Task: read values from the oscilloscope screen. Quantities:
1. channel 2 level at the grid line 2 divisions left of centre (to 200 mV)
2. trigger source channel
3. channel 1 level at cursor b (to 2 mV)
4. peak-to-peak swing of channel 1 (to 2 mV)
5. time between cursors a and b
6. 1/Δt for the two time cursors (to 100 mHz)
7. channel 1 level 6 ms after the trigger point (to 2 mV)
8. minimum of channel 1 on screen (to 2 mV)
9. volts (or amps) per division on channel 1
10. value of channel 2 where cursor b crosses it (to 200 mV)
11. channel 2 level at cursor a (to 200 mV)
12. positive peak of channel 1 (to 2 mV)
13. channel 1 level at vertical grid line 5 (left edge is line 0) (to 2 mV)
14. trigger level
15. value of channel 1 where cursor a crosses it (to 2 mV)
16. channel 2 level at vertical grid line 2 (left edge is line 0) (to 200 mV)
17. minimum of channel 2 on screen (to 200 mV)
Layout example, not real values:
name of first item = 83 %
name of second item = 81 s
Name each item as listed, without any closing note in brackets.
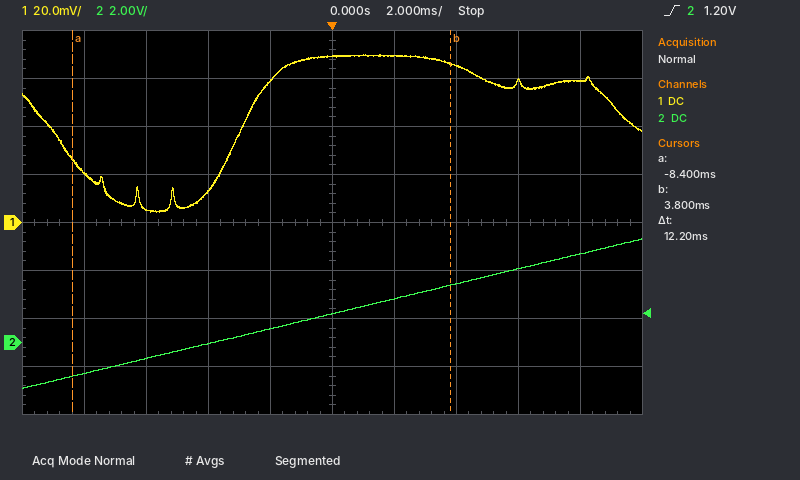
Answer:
channel 2 level at the grid line 2 divisions left of centre = 0.0 V
trigger source channel = channel 2
channel 1 level at cursor b = 66 mV
peak-to-peak swing of channel 1 = 66 mV
time between cursors a and b = 12.2 ms
1/Δt for the two time cursors = 82.0 Hz
channel 1 level 6 ms after the trigger point = 58 mV
minimum of channel 1 on screen = 4 mV
volts (or amps) per division on channel 1 = 20 mV
value of channel 2 where cursor b crosses it = 2.4 V
channel 2 level at cursor a = -1.4 V
positive peak of channel 1 = 70 mV
channel 1 level at vertical grid line 5 (left edge is line 0) = 70 mV
trigger level = 1.20 V
value of channel 1 where cursor a crosses it = 26 mV
channel 2 level at vertical grid line 2 (left edge is line 0) = -600 mV
minimum of channel 2 on screen = -2.0 V
